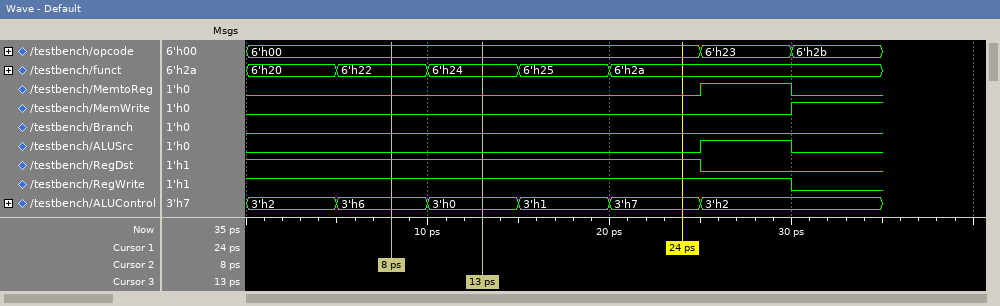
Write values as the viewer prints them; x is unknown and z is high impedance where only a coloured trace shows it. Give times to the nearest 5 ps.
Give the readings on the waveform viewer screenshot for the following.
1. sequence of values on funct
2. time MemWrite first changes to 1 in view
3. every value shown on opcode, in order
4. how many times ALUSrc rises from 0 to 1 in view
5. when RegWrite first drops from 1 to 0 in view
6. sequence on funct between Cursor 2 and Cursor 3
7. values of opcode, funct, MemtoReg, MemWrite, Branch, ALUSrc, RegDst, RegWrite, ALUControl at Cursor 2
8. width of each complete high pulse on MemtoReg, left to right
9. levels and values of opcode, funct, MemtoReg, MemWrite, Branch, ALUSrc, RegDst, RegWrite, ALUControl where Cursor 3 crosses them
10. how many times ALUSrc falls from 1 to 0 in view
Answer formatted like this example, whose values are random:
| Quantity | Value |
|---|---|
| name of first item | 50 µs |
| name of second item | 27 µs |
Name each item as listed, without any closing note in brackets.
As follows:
| Quantity | Value |
|---|---|
| sequence of values on funct | 6'h20, 6'h22, 6'h24, 6'h25, 6'h2a |
| time MemWrite first changes to 1 in view | 30 ps |
| every value shown on opcode, in order | 6'h00, 6'h23, 6'h2b |
| how many times ALUSrc rises from 0 to 1 in view | 1 |
| when RegWrite first drops from 1 to 0 in view | 30 ps |
| sequence on funct between Cursor 2 and Cursor 3 | 6'h22, 6'h24 |
| values of opcode, funct, MemtoReg, MemWrite, Branch, ALUSrc, RegDst, RegWrite, ALUControl at Cursor 2 | opcode=6'h00, funct=6'h22, MemtoReg=0, MemWrite=0, Branch=0, ALUSrc=0, RegDst=1, RegWrite=1, ALUControl=3'h6 |
| width of each complete high pulse on MemtoReg, left to right | 5 ps |
| levels and values of opcode, funct, MemtoReg, MemWrite, Branch, ALUSrc, RegDst, RegWrite, ALUControl where Cursor 3 crosses them | opcode=6'h00, funct=6'h24, MemtoReg=0, MemWrite=0, Branch=0, ALUSrc=0, RegDst=1, RegWrite=1, ALUControl=3'h0 |
| how many times ALUSrc falls from 1 to 0 in view | 1 |
